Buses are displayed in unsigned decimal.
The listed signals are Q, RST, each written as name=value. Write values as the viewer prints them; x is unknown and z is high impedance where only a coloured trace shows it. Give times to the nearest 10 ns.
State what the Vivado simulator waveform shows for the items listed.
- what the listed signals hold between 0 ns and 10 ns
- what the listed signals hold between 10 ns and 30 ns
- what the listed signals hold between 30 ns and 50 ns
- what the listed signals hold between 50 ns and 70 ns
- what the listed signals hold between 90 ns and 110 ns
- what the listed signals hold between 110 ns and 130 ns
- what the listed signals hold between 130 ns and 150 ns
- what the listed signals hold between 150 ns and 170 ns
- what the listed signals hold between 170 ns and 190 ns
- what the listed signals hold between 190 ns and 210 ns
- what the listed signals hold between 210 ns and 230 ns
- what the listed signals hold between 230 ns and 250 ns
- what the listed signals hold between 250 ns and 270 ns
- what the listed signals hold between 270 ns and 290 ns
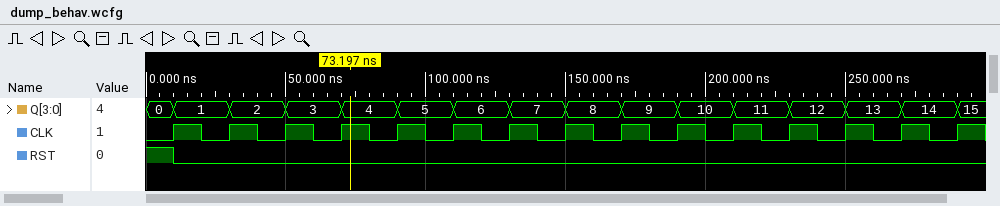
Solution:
Q=0, RST=1
Q=1, RST=0
Q=2, RST=0
Q=3, RST=0
Q=5, RST=0
Q=6, RST=0
Q=7, RST=0
Q=8, RST=0
Q=9, RST=0
Q=10, RST=0
Q=11, RST=0
Q=12, RST=0
Q=13, RST=0
Q=14, RST=0
